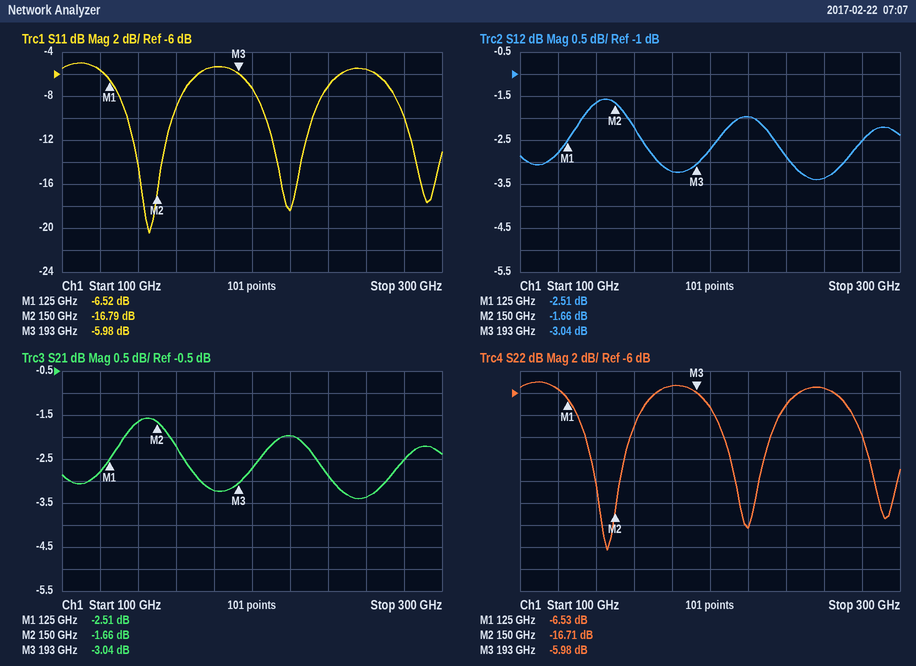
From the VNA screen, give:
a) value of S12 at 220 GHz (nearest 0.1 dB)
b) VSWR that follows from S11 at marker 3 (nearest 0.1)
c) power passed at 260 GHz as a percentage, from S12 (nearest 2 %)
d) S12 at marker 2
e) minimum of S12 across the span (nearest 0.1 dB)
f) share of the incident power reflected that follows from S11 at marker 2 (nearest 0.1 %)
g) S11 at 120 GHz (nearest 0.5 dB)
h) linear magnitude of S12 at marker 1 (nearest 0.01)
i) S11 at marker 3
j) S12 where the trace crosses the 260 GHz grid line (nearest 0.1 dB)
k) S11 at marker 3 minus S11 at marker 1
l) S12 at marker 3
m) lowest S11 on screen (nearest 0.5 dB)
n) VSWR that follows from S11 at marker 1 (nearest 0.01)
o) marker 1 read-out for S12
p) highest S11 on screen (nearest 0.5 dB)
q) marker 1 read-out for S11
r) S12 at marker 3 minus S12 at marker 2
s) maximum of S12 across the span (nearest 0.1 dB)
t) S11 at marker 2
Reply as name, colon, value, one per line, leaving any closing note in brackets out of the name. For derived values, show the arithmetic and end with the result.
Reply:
value of S12 at 220 GHz: -2.0 dB
VSWR that follows from S11 at marker 3: (1 + 0.5023)/(1 − 0.5023) ≈ 3.0
power passed at 260 GHz as a percentage, from S12: 10^(-3.4/10) ≈ 46 %
S12 at marker 2: -1.66 dB
minimum of S12 across the span: -3.4 dB
share of the incident power reflected that follows from S11 at marker 2: 10^(-16.79/10) ≈ 2.1 %
S11 at 120 GHz: -5.5 dB
linear magnitude of S12 at marker 1: 10^(-2.51/20) ≈ 0.75
S11 at marker 3: -5.98 dB
S12 where the trace crosses the 260 GHz grid line: -3.4 dB
S11 at marker 3 minus S11 at marker 1: -5.98 − (-6.52) = 0.54 dB
S12 at marker 3: -3.04 dB
lowest S11 on screen: -20.5 dB
VSWR that follows from S11 at marker 1: (1 + 0.4721)/(1 − 0.4721) ≈ 2.79
marker 1 read-out for S12: -2.51 dB
highest S11 on screen: -5.0 dB
marker 1 read-out for S11: -6.52 dB
S12 at marker 3 minus S12 at marker 2: -3.04 − (-1.66) = -1.38 dB
maximum of S12 across the span: -1.6 dB
S11 at marker 2: -16.79 dB
